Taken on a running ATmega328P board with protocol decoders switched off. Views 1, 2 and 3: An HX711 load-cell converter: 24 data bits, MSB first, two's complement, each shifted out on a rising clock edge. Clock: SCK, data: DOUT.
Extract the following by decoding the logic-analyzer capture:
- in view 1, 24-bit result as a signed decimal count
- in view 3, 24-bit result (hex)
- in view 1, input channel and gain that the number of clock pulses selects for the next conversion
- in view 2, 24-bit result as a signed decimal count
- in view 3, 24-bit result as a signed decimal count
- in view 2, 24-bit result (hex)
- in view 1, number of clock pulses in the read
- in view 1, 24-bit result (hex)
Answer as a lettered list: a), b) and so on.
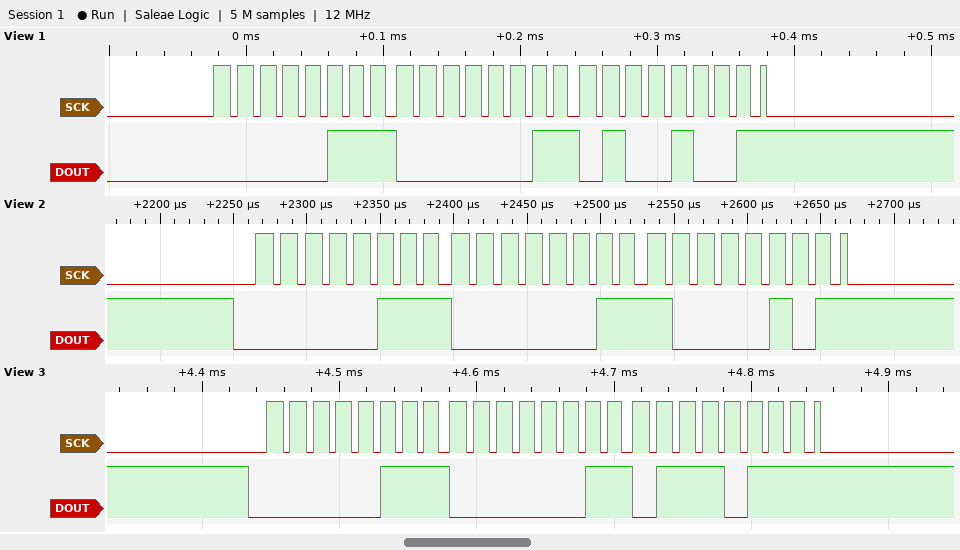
a) 459593
b) 0x070377
c) channel A, gain 128
d) 459653
e) 459639
f) 0x070385
g) 25
h) 0x070349
